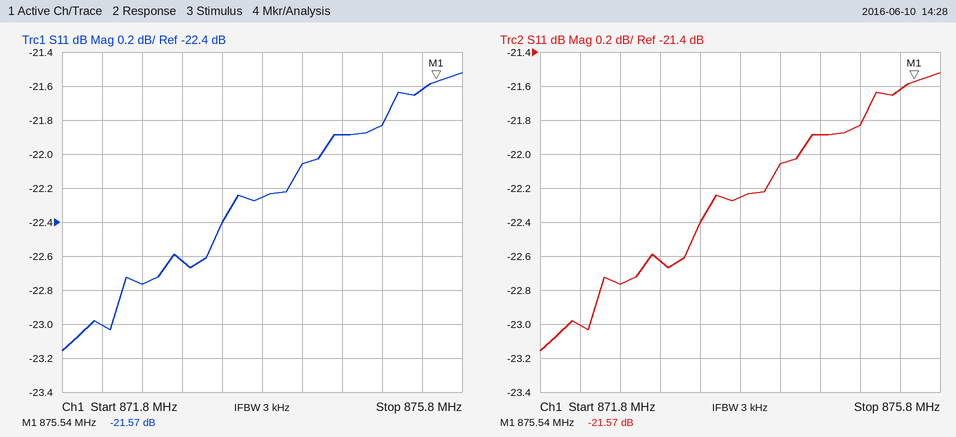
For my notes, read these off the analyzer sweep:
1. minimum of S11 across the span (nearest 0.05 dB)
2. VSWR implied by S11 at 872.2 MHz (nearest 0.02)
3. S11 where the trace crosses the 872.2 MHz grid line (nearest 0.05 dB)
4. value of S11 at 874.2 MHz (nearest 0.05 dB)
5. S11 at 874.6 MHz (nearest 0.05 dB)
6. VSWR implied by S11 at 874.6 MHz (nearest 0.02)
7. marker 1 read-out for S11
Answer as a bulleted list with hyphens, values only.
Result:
- -23.15 dB
- 1.16
- -23.00 dB
- -22.05 dB
- -21.90 dB
- 1.18
- -21.57 dB
